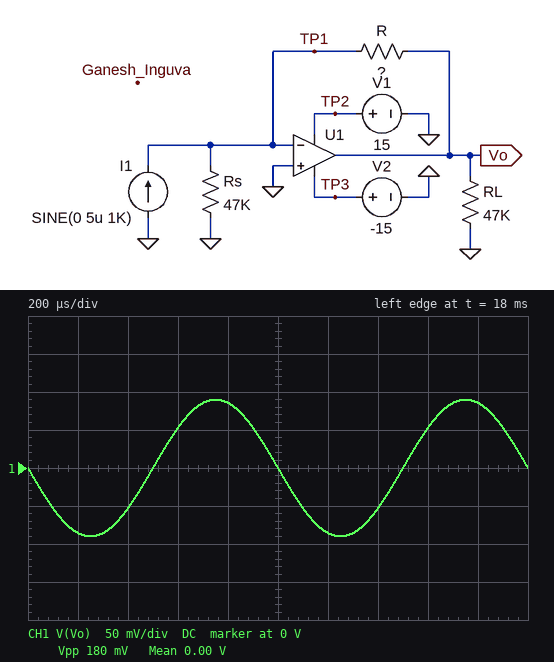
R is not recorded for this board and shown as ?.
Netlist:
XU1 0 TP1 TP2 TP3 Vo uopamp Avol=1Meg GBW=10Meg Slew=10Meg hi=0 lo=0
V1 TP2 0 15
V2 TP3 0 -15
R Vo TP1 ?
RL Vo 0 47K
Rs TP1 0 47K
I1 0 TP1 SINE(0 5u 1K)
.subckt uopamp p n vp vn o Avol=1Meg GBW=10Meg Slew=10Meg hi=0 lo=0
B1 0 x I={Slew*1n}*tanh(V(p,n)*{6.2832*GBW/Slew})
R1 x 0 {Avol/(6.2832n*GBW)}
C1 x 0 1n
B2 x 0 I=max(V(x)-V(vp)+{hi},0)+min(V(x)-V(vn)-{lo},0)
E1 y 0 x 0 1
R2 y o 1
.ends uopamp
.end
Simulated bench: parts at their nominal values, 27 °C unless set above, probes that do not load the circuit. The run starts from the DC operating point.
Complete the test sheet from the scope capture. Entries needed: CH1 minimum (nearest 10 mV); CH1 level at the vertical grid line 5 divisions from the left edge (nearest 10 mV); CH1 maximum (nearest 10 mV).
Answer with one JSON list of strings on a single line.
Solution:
["-90 mV", "0 V", "90 mV"]
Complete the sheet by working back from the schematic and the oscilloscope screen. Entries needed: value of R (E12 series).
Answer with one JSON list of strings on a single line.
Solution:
["18 kΩ"]
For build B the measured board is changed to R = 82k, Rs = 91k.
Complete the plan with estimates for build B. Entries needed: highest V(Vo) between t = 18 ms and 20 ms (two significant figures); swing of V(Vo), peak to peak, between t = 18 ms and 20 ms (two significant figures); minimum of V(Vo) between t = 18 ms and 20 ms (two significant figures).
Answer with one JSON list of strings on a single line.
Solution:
["410 mV", "820 mV", "-410 mV"]
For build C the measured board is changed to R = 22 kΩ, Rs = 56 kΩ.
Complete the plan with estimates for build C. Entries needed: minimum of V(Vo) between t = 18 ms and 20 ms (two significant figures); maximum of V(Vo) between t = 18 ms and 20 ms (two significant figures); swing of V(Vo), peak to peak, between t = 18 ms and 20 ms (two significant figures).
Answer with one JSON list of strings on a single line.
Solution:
["-110 mV", "110 mV", "220 mV"]
